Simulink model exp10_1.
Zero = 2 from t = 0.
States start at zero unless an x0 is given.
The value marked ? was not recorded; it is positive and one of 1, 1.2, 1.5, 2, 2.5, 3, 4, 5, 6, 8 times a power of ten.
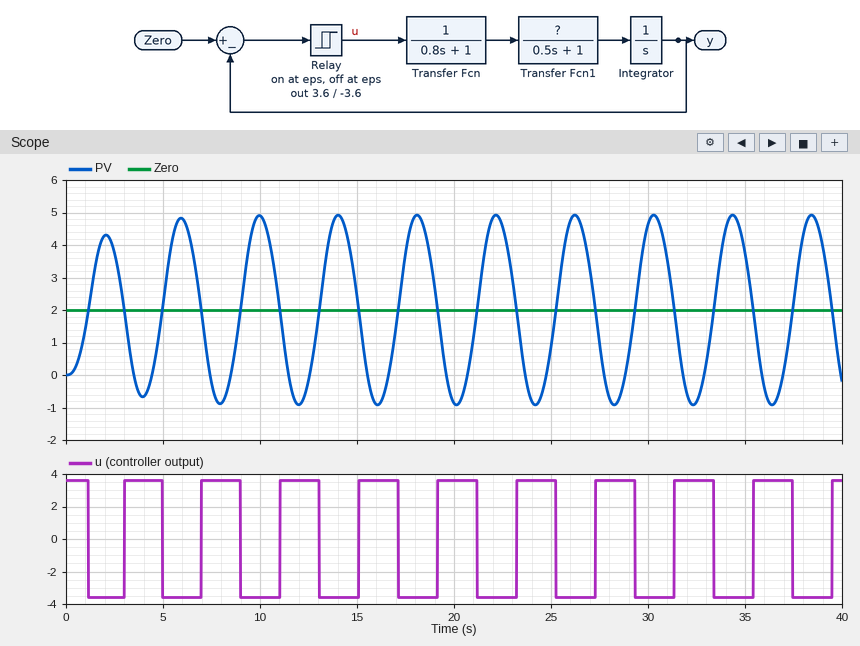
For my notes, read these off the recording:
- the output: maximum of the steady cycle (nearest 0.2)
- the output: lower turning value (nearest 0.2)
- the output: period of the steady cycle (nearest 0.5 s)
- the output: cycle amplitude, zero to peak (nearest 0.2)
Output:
5.0
-1.0
4.0 s
3.0
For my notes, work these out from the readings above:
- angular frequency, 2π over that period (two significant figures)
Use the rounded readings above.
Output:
1.6 rad/s
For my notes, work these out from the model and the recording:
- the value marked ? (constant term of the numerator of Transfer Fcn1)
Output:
2
